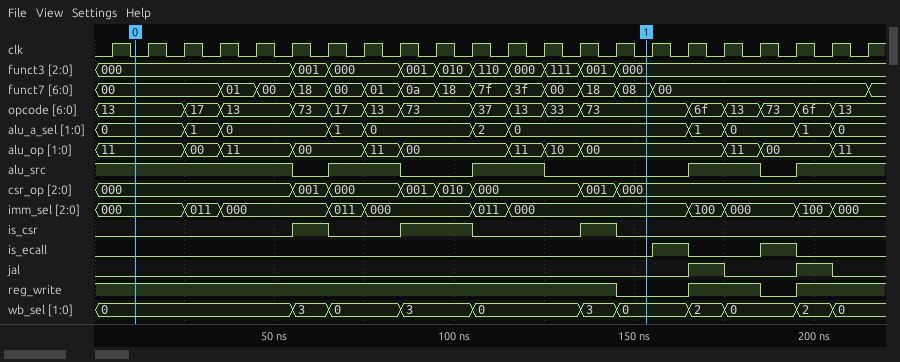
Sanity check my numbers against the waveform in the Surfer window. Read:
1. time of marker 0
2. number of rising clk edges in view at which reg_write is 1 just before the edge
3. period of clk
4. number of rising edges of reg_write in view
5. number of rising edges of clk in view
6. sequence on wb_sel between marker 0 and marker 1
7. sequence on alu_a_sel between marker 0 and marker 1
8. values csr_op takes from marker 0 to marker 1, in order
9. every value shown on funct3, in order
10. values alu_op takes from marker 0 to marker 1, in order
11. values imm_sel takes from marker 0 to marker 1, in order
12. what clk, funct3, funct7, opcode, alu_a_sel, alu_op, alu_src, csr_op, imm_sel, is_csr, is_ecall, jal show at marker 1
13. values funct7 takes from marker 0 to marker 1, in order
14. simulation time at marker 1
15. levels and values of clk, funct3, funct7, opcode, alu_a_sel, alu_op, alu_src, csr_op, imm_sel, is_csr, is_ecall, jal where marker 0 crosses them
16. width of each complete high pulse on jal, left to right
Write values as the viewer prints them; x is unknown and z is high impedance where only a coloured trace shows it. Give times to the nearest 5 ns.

10 ns
19
10 ns
2
22
0, 3, 0, 3, 0, 3, 0
0, 1, 0, 1, 0, 2, 0
000, 001, 000, 001, 010, 000, 001, 000
000, 001, 000, 001, 010, 110, 000, 111, 001, 000
11, 00, 11, 00, 11, 00, 11, 10, 00
000, 011, 000, 011, 000, 011, 000
clk=0, funct3=000, funct7=08, opcode=73, alu_a_sel=0, alu_op=00, alu_src=0, csr_op=000, imm_sel=000, is_csr=0, is_ecall=0, jal=0
00, 01, 00, 18, 00, 01, 0a, 18, 7f, 3f, 00, 18, 08
155 ns
clk=0, funct3=000, funct7=00, opcode=13, alu_a_sel=0, alu_op=11, alu_src=1, csr_op=000, imm_sel=000, is_csr=0, is_ecall=0, jal=0
10 ns, 10 ns
